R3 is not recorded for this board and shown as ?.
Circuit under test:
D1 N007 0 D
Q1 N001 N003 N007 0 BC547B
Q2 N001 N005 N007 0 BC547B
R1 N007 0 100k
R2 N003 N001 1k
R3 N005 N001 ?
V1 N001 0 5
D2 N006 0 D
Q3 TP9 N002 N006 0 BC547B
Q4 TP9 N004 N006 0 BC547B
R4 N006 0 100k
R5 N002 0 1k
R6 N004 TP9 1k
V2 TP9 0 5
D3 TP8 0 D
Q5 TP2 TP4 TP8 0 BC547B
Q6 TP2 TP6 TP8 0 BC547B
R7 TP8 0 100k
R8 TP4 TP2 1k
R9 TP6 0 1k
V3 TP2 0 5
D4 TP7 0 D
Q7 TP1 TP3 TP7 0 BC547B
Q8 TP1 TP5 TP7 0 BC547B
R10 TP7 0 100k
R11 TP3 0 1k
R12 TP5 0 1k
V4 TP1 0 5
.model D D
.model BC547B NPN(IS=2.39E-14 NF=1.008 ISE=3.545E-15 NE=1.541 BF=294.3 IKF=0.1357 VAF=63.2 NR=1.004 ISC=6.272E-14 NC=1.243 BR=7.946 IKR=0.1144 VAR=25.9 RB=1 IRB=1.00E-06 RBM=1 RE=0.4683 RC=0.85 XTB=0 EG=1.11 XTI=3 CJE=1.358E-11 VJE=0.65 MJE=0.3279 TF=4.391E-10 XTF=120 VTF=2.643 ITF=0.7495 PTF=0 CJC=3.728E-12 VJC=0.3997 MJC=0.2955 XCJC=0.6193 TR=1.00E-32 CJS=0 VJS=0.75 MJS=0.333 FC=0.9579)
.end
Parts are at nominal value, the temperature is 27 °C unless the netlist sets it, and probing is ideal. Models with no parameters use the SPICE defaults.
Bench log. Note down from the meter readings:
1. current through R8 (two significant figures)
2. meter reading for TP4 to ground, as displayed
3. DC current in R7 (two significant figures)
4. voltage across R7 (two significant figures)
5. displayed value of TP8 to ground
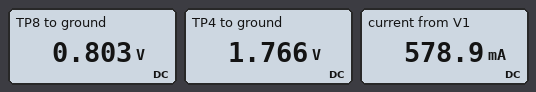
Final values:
3.2 mA
1.766 V
8.0 µA
800 mV
0.803 V
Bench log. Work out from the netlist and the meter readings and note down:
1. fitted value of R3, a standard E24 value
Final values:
1.2 kΩ
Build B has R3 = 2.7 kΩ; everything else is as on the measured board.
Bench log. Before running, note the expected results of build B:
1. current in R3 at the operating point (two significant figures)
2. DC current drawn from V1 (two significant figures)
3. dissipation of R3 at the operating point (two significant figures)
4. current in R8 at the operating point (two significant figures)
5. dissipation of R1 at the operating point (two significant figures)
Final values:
1.2 mA
470 mA
4.1 mW
3.2 mA
6.6 µW
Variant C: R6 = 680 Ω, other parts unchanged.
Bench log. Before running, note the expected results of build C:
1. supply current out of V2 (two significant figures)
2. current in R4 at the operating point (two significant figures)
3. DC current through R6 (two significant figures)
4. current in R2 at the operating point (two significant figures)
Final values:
380 mA
8.1 µA
4.7 mA
3.2 mA
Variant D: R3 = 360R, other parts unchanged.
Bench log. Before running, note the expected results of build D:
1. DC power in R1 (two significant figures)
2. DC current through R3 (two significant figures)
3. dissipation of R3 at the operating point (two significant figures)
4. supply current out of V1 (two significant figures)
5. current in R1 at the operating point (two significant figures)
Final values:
6.9 µW
8.5 mA
26 mW
840 mA
8.3 µA
